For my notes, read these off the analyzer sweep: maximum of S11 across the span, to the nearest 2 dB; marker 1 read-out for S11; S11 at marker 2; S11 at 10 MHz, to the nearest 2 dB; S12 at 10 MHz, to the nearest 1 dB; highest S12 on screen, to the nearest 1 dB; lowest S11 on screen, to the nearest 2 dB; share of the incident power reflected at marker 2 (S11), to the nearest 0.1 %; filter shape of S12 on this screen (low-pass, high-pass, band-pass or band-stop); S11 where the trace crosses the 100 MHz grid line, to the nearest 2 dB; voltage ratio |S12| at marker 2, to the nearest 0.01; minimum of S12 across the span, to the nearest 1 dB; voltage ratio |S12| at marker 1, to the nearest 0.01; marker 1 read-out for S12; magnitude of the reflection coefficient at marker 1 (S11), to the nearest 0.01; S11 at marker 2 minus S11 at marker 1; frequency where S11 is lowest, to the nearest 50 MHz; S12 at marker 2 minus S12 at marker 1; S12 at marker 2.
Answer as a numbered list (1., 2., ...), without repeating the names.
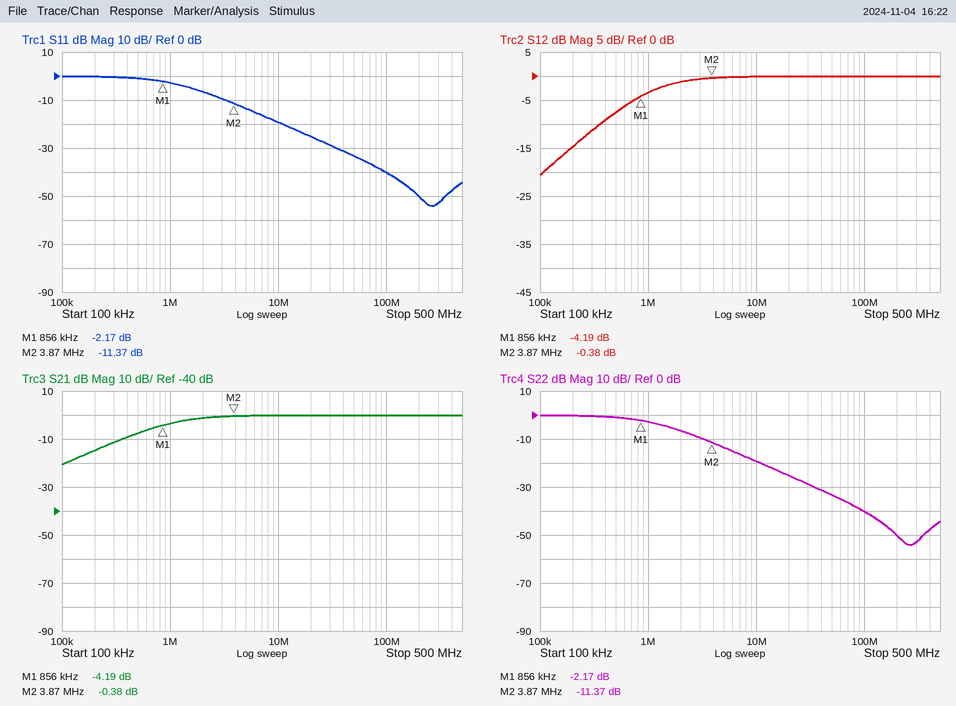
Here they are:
1. 0 dB
2. -2.17 dB
3. -11.37 dB
4. -20 dB
5. 0 dB
6. 0 dB
7. -54 dB
8. 7.3 %
9. high-pass
10. -40 dB
11. 0.96
12. -21 dB
13. 0.62
14. -4.19 dB
15. 0.78
16. -9.20 dB
17. 250 MHz
18. 3.81 dB
19. -0.38 dB
